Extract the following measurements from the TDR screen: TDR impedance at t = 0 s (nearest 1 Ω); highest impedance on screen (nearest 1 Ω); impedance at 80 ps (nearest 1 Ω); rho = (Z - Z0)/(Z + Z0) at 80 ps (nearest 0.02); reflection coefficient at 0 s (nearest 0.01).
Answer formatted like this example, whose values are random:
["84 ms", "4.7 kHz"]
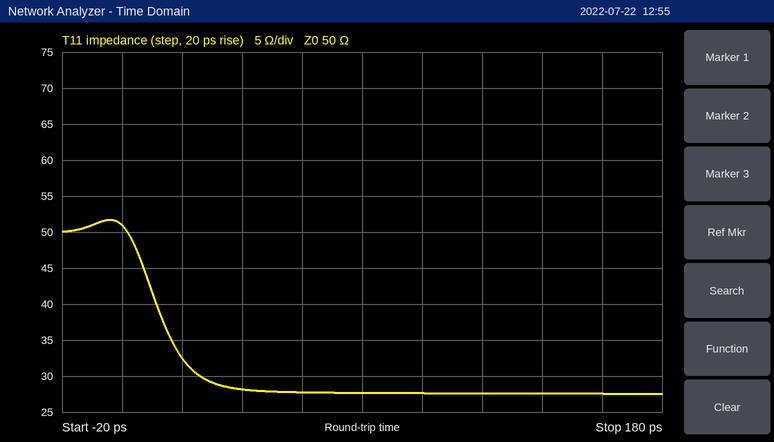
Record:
["51 Ω", "52 Ω", "28 Ω", "-0.28", "+0.01"]
